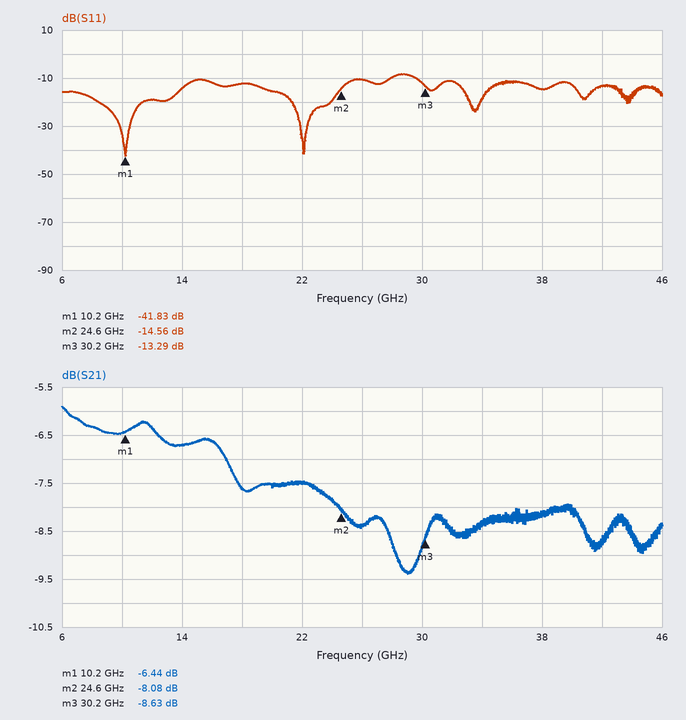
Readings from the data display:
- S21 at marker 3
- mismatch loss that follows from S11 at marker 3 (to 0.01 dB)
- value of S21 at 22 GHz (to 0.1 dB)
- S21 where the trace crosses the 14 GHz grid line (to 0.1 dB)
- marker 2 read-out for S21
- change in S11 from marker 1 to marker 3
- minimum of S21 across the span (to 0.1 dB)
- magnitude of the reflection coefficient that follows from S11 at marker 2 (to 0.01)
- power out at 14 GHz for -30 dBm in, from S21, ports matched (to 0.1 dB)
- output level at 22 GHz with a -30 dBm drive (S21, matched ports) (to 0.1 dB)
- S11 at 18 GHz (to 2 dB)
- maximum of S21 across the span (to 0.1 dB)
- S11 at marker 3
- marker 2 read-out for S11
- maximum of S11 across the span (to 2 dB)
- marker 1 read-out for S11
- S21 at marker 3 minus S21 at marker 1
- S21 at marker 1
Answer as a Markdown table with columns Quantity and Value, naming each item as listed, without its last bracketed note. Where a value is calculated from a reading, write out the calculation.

| Quantity | Value |
|---|---|
| S21 at marker 3 | -8.63 dB |
| mismatch loss that follows from S11 at marker 3 | −10 log10(1 − 10^(-13.29/10)) ≈ 0.21 dB |
| value of S21 at 22 GHz | -7.5 dB |
| S21 where the trace crosses the 14 GHz grid line | -6.7 dB |
| marker 2 read-out for S21 | -8.08 dB |
| change in S11 from marker 1 to marker 3 | -13.29 − (-41.83) = 28.54 dB |
| minimum of S21 across the span | -9.4 dB |
| magnitude of the reflection coefficient that follows from S11 at marker 2 | 10^(-14.56/20) ≈ 0.19 |
| power out at 14 GHz for -30 dBm in, from S21, ports matched | -30 dBm + (-6.7 dB) = -36.7 dBm |
| output level at 22 GHz with a -30 dBm drive (S21, matched ports) | -30 dBm + (-7.5 dB) = -37.5 dBm |
| S11 at 18 GHz | -12 dB |
| maximum of S21 across the span | -5.9 dB |
| S11 at marker 3 | -13.29 dB |
| marker 2 read-out for S11 | -14.56 dB |
| maximum of S11 across the span | -8 dB |
| marker 1 read-out for S11 | -41.83 dB |
| S21 at marker 3 minus S21 at marker 1 | -8.63 − (-6.44) = -2.19 dB |
| S21 at marker 1 | -6.44 dB |
